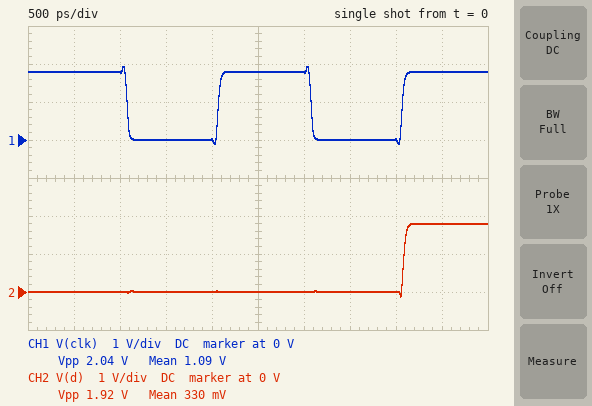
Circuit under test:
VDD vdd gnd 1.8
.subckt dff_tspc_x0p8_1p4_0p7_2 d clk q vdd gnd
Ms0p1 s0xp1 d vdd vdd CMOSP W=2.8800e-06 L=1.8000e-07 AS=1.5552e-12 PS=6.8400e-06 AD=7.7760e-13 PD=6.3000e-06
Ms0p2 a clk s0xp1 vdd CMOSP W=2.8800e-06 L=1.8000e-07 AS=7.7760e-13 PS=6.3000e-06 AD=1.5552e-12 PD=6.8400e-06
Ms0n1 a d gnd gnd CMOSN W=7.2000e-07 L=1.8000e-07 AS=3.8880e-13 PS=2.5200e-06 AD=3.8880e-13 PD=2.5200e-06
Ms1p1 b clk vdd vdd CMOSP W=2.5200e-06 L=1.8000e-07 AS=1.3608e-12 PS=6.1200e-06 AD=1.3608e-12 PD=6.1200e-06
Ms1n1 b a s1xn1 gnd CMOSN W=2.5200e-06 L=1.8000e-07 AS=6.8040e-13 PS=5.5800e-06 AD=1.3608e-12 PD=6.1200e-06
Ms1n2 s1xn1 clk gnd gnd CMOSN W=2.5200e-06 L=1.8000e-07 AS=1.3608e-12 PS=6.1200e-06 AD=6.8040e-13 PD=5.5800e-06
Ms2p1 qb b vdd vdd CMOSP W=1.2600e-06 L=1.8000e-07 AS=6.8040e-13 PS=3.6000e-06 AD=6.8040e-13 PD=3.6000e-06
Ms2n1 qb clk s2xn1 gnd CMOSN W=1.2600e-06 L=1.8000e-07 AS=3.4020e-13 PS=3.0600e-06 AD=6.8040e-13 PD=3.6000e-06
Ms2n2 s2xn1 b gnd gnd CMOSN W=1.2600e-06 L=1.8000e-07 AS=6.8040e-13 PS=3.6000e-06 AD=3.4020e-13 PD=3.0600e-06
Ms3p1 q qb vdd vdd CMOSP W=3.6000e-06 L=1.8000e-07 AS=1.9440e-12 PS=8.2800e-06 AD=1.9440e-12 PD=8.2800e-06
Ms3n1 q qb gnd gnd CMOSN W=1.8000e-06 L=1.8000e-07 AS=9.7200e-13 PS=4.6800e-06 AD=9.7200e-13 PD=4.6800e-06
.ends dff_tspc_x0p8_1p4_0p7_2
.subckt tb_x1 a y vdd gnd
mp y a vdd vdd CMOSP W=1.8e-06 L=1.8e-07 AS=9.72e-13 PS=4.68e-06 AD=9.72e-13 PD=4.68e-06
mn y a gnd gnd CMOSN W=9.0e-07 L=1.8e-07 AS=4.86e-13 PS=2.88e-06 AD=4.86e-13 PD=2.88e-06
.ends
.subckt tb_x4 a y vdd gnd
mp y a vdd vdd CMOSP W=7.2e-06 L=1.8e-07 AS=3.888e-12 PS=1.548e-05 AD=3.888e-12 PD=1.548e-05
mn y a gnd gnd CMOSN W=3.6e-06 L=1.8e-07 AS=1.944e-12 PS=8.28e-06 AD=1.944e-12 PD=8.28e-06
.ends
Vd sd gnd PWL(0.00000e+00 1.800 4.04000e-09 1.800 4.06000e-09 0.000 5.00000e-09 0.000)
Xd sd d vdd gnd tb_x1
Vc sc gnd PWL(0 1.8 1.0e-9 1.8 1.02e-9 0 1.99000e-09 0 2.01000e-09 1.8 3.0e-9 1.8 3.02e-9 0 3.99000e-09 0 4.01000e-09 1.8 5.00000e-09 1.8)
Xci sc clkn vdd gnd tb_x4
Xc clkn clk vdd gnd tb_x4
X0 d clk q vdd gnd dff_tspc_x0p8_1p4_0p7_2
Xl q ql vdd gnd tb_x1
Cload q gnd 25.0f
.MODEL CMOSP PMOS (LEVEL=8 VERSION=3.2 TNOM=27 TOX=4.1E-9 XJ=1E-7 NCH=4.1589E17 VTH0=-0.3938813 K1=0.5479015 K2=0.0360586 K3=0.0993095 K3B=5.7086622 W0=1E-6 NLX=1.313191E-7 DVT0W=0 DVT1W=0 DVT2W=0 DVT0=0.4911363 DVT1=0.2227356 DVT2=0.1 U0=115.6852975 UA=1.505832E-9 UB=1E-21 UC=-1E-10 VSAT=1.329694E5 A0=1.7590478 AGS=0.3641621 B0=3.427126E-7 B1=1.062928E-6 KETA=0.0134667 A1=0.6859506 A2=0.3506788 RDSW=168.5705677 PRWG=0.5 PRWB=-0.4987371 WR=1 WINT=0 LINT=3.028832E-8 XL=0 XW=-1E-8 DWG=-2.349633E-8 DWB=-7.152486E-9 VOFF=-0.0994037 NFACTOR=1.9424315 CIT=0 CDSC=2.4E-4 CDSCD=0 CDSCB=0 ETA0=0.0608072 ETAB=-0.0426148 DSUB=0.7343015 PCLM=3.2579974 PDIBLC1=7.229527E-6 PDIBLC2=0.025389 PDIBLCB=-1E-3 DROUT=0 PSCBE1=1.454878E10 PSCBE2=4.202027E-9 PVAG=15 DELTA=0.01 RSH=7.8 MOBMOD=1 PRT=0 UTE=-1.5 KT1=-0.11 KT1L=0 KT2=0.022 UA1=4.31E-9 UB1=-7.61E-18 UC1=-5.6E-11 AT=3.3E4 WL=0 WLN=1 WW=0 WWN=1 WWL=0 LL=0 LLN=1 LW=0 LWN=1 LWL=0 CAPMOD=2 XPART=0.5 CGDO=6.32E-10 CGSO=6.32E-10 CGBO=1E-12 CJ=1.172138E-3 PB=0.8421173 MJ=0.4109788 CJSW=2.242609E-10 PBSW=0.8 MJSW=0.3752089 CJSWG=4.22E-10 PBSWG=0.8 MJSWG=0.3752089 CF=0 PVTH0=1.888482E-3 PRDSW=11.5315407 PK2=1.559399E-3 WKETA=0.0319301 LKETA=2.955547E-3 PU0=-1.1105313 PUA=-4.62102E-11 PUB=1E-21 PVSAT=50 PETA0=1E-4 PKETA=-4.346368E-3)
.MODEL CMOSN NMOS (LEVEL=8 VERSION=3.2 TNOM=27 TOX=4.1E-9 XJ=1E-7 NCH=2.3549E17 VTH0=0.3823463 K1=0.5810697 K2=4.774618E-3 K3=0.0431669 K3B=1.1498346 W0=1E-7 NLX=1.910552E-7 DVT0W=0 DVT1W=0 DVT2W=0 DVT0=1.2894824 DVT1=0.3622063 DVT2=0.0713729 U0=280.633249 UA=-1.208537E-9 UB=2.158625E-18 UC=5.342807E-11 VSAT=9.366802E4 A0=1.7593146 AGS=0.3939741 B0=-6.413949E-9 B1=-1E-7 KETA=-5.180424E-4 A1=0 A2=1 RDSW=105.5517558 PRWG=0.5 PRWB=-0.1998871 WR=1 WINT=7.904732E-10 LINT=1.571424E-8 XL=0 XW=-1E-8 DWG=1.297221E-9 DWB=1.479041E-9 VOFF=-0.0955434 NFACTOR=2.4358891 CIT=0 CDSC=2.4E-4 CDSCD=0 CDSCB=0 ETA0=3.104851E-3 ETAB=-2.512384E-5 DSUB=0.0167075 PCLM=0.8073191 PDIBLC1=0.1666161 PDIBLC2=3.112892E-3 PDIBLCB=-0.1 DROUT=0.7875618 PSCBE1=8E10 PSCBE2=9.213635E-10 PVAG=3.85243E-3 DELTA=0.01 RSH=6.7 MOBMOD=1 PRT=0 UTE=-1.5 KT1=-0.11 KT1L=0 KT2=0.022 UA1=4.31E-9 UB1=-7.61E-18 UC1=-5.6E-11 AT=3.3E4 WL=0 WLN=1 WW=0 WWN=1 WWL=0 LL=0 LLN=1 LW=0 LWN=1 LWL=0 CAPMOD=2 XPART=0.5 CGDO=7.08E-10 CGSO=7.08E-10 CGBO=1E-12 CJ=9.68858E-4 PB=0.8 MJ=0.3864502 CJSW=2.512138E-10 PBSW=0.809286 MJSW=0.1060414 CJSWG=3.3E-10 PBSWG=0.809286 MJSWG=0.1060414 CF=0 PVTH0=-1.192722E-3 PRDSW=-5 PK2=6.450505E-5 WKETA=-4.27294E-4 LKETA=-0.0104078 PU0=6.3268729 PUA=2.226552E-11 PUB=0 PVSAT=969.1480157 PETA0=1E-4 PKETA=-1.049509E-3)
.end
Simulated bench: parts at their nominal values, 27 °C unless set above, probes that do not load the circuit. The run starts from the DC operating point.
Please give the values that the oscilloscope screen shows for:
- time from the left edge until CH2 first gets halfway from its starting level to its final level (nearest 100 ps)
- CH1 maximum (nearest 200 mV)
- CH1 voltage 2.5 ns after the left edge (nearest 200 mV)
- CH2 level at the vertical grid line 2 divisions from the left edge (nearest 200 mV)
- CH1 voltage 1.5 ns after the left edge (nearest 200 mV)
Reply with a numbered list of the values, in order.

1. 4.1 ns
2. 2.0 V
3. 1.8 V
4. 0 V
5. 0 V
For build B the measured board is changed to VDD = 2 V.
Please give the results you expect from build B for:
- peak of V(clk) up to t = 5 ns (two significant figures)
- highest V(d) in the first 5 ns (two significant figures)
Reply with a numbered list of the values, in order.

1. 2.1 V
2. 2.0 V
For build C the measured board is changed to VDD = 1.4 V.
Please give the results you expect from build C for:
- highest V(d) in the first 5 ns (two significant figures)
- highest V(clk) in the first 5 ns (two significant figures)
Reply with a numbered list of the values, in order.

1. 1.4 V
2. 1.5 V
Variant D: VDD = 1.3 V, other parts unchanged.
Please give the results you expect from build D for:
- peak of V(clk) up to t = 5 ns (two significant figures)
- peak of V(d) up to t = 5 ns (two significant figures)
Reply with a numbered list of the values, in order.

1. 1.4 V
2. 1.3 V
